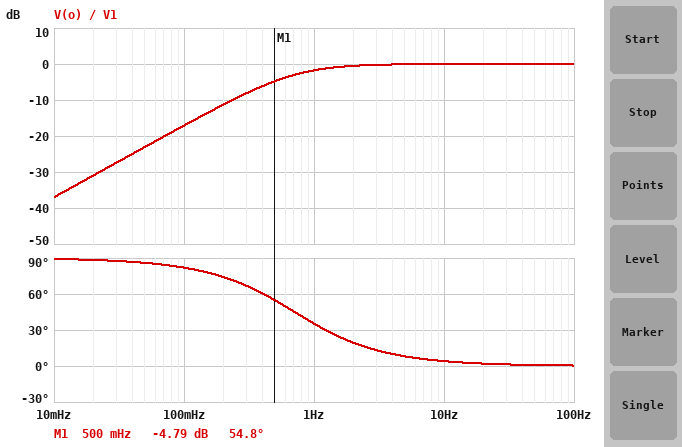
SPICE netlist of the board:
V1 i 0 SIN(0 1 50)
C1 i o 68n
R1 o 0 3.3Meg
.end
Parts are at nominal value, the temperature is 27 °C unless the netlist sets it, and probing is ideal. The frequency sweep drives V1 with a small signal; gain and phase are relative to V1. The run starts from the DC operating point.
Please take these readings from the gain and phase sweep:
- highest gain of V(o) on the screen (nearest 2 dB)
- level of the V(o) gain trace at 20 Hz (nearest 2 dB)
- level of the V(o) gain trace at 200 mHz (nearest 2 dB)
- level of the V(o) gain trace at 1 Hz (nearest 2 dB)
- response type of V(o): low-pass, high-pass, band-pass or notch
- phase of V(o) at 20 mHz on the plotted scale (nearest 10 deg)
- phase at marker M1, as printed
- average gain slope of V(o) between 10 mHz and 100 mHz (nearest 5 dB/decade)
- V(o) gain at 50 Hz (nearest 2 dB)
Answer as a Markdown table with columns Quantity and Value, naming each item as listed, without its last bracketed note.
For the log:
| Quantity | Value |
|---|---|
| highest gain of V(o) on the screen | 0 dB |
| level of the V(o) gain trace at 20 Hz | 0 dB |
| level of the V(o) gain trace at 200 mHz | -12 dB |
| level of the V(o) gain trace at 1 Hz | -2 dB |
| response type of V(o): low-pass, high-pass, band-pass or notch | high-pass |
| phase of V(o) at 20 mHz on the plotted scale | 90 deg |
| phase at marker M1, as printed | 54.8 deg |
| average gain slope of V(o) between 10 mHz and 100 mHz | 20 dB/decade |
| V(o) gain at 50 Hz | 0 dB |
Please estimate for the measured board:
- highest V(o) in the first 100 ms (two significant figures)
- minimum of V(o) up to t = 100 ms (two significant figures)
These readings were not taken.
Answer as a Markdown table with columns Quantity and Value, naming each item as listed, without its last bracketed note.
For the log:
| Quantity | Value |
|---|---|
| highest V(o) in the first 100 ms | 990 mV |
| minimum of V(o) up to t = 100 ms | -1.0 V |
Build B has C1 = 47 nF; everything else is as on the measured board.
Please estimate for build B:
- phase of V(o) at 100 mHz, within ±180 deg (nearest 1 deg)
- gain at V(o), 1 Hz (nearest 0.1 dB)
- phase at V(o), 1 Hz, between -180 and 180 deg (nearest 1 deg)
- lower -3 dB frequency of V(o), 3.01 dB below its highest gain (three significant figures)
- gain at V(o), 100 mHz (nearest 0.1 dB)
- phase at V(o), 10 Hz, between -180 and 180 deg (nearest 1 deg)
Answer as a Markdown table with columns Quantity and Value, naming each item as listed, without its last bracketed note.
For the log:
| Quantity | Value |
|---|---|
| phase of V(o) at 100 mHz, within ±180 deg | 84 deg |
| gain at V(o), 1 Hz | -3.1 dB |
| phase at V(o), 1 Hz, between -180 and 180 deg | 46 deg |
| lower -3 dB frequency of V(o), 3.01 dB below its highest gain | 1.03 Hz |
| gain at V(o), 100 mHz | -20.3 dB |
| phase at V(o), 10 Hz, between -180 and 180 deg | 6 deg |
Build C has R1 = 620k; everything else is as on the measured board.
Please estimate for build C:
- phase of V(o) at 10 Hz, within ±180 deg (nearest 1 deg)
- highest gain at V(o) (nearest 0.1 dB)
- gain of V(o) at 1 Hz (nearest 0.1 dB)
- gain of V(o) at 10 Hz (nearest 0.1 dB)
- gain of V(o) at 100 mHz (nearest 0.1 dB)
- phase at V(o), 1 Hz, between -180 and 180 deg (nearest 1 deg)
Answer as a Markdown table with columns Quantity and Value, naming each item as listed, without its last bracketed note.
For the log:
| Quantity | Value |
|---|---|
| phase of V(o) at 10 Hz, within ±180 deg | 21 deg |
| highest gain at V(o) | 0 dB |
| gain of V(o) at 1 Hz | -11.8 dB |
| gain of V(o) at 10 Hz | -0.6 dB |
| gain of V(o) at 100 mHz | -31.5 dB |
| phase at V(o), 1 Hz, between -180 and 180 deg | 75 deg |
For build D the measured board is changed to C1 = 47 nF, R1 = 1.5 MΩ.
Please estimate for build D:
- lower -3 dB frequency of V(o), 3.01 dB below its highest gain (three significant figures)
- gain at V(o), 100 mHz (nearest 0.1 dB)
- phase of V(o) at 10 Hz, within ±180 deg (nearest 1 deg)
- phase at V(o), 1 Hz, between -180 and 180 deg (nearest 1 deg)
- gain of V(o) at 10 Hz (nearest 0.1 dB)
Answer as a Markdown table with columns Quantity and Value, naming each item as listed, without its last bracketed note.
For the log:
| Quantity | Value |
|---|---|
| lower -3 dB frequency of V(o), 3.01 dB below its highest gain | 2.26 Hz |
| gain at V(o), 100 mHz | -27.1 dB |
| phase of V(o) at 10 Hz, within ±180 deg | 13 deg |
| phase at V(o), 1 Hz, between -180 and 180 deg | 66 deg |
| gain of V(o) at 10 Hz | -0.2 dB |
